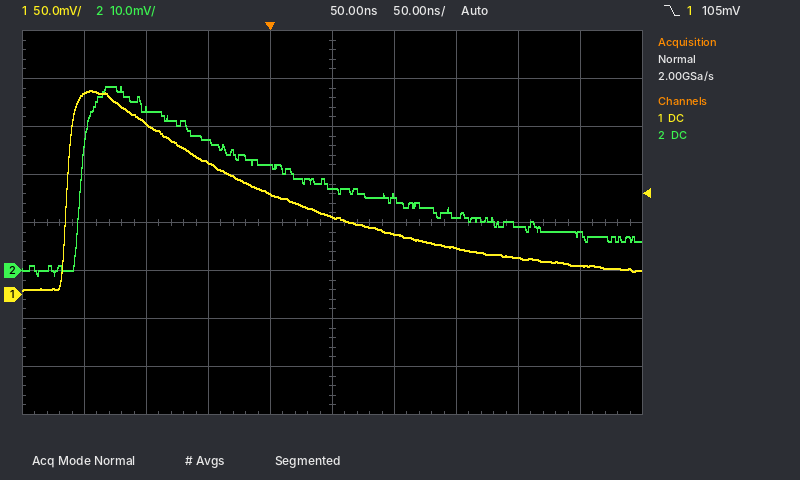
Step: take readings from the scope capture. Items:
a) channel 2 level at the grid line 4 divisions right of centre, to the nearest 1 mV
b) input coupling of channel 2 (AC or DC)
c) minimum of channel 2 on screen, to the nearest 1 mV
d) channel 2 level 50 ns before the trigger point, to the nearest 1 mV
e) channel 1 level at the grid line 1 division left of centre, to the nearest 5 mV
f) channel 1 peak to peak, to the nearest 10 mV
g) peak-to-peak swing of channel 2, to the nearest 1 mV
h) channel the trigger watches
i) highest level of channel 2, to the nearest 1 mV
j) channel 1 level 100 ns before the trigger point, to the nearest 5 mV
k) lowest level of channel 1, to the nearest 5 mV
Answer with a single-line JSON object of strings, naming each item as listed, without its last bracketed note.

{"channel 2 level at the grid line 4 divisions right of centre, to the nearest 1 mV": "8 mV", "input coupling of channel 2": "DC", "minimum of channel 2 on screen, to the nearest 1 mV": "-1 mV", "channel 2 level 50 ns before the trigger point, to the nearest 1 mV": "27 mV", "channel 1 level at the grid line 1 division left of centre, to the nearest 5 mV": "105 mV", "channel 1 peak to peak, to the nearest 10 mV": "210 mV", "peak-to-peak swing of channel 2, to the nearest 1 mV": "39 mV", "channel the trigger watches": "channel 1", "highest level of channel 2, to the nearest 1 mV": "38 mV", "channel 1 level 100 ns before the trigger point, to the nearest 5 mV": "180 mV", "lowest level of channel 1, to the nearest 5 mV": "5 mV"}
